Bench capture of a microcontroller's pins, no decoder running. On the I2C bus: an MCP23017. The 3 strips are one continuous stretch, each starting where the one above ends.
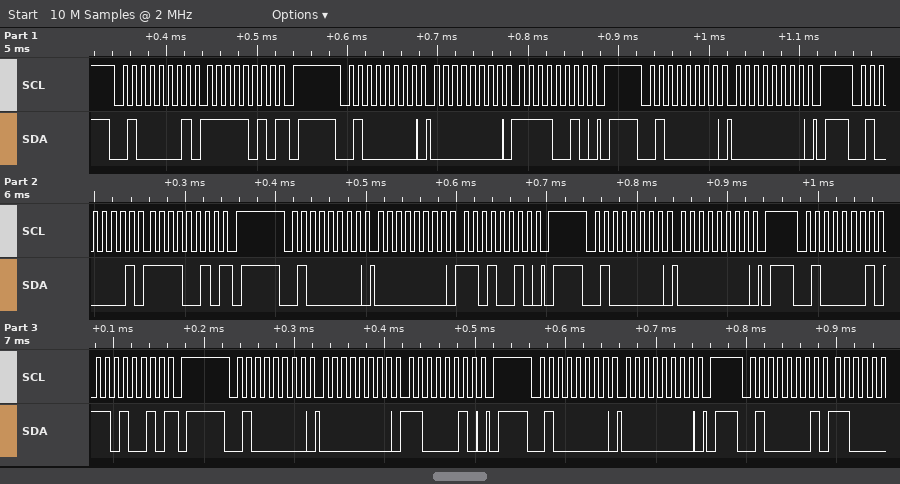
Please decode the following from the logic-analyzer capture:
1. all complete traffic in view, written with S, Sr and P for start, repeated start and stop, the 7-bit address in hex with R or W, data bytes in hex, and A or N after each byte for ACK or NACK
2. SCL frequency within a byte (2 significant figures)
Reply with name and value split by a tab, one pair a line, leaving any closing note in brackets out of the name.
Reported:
all complete traffic in view, written with S, Sr and P for start, repeated start and stop, the 7-bit address in hex with R or W, data bytes in hex, and A or N after each byte for ACK or NACK	S 20R A FA N P S 20W A 00 A F2 A P S 20W A 00 A P S 20R A F2 N P S 20W A 00 A D2 A P S 20W A 00 A P S 20R A D2 N P S 20W A 00 A C2 A P S 20W A 00 A P S 20R A
SCL frequency within a byte	100 kHz
